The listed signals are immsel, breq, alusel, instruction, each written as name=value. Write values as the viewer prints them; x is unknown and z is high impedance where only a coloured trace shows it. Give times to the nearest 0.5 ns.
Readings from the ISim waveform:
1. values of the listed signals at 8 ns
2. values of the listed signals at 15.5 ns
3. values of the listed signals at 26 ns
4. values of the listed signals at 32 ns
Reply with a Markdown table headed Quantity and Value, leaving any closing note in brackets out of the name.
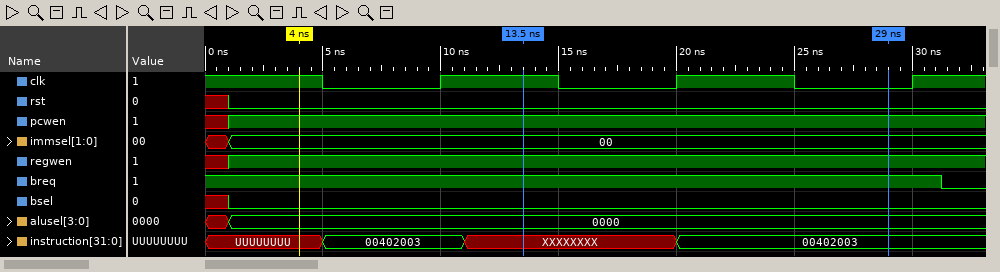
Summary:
| Quantity | Value |
|---|---|
| values of the listed signals at 8 ns | immsel=00, breq=1, alusel=0000, instruction=00402003 |
| values of the listed signals at 15.5 ns | immsel=00, breq=1, alusel=0000, instruction=XXXXXXXX |
| values of the listed signals at 26 ns | immsel=00, breq=1, alusel=0000, instruction=00402003 |
| values of the listed signals at 32 ns | immsel=00, breq=0, alusel=0000, instruction=00402003 |
